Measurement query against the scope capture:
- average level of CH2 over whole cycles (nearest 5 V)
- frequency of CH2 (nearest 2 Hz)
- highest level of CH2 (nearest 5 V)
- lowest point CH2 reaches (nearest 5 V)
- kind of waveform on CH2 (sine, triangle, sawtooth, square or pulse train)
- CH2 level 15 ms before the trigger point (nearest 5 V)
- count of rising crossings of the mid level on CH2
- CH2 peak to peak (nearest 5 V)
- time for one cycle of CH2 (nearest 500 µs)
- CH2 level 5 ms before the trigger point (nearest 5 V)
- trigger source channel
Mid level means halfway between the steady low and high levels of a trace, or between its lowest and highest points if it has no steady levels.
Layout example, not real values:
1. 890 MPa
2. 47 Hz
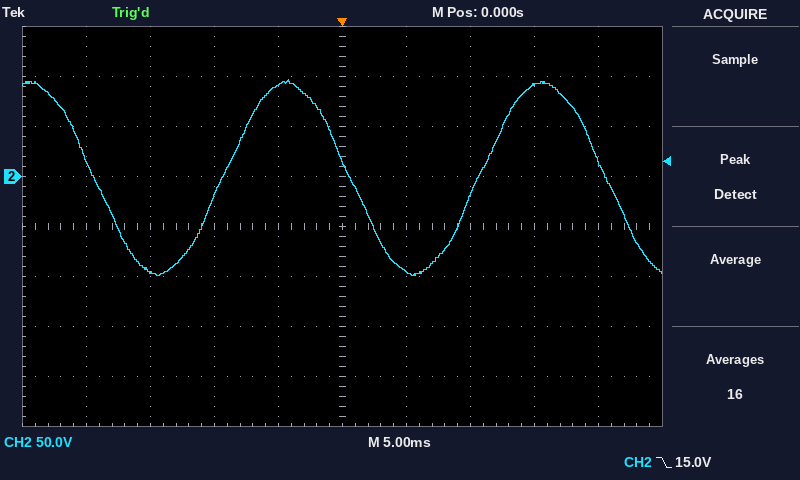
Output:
1. 0 V
2. 50 Hz
3. 95 V
4. -100 V
5. sine
6. -95 V
7. 2
8. 195 V
9. 20.0 ms
10. 90 V
11. CH2
